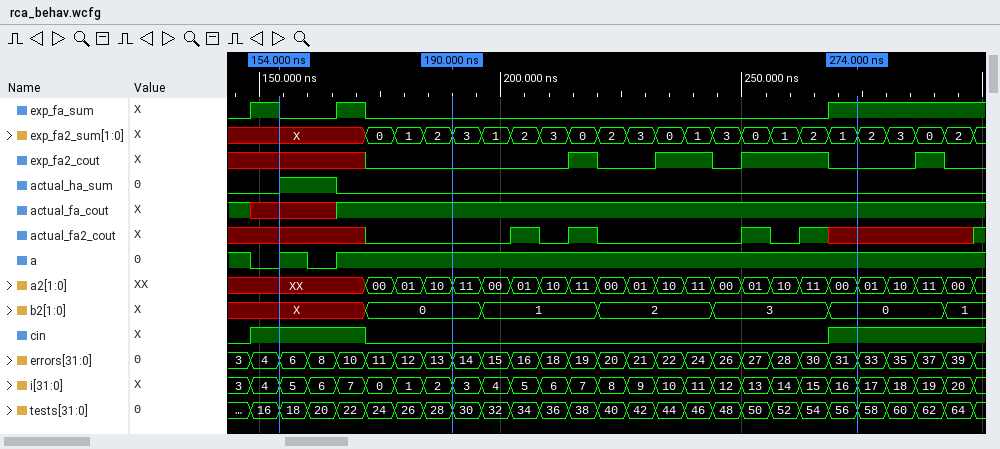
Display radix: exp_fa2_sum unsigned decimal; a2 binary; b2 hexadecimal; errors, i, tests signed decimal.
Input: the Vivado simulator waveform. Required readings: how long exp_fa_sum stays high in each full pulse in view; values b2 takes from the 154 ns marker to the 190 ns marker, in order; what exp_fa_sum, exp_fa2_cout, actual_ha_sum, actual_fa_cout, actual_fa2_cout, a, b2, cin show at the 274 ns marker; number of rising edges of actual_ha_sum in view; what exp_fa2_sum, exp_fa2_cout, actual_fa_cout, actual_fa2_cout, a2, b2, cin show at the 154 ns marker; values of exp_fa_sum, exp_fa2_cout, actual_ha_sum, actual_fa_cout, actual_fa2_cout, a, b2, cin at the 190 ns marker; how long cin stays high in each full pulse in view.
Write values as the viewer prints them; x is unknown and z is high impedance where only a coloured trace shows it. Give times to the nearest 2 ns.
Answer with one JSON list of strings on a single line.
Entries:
["6 ns, 6 ns", "X, 0", "exp_fa_sum=1, exp_fa2_cout=0, actual_ha_sum=0, actual_fa_cout=1, actual_fa2_cout=x, a=1, b2=0, cin=1", "1", "exp_fa2_sum=X, exp_fa2_cout=x, actual_fa_cout=x, actual_fa2_cout=x, a2=XX, b2=X, cin=1", "exp_fa_sum=0, exp_fa2_cout=0, actual_ha_sum=0, actual_fa_cout=1, actual_fa2_cout=0, a=1, b2=0, cin=0", "24 ns"]
